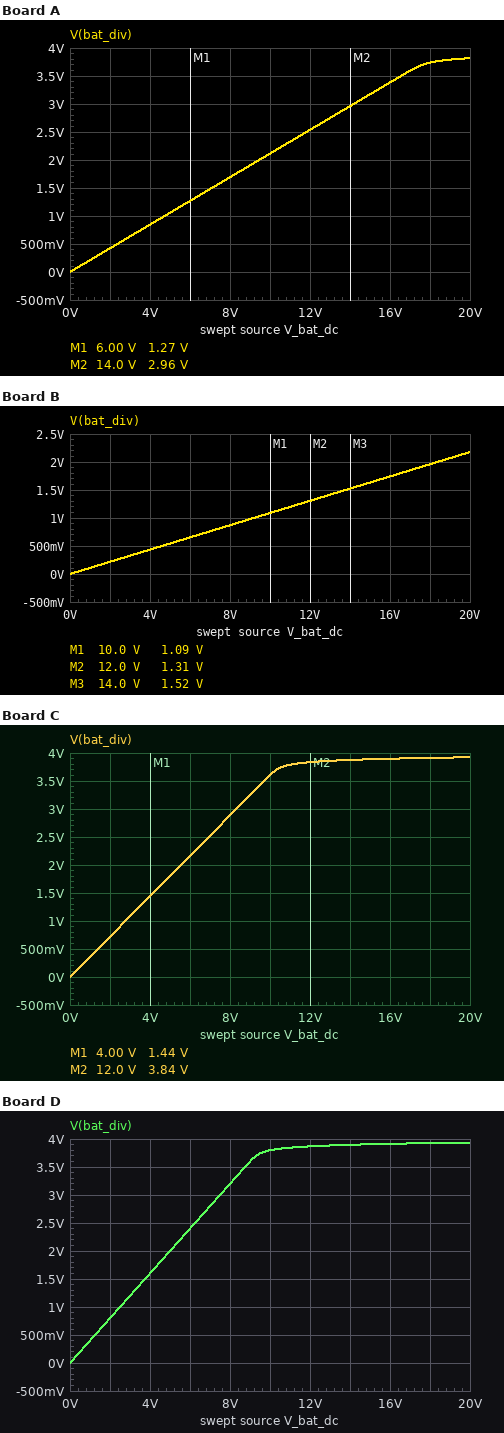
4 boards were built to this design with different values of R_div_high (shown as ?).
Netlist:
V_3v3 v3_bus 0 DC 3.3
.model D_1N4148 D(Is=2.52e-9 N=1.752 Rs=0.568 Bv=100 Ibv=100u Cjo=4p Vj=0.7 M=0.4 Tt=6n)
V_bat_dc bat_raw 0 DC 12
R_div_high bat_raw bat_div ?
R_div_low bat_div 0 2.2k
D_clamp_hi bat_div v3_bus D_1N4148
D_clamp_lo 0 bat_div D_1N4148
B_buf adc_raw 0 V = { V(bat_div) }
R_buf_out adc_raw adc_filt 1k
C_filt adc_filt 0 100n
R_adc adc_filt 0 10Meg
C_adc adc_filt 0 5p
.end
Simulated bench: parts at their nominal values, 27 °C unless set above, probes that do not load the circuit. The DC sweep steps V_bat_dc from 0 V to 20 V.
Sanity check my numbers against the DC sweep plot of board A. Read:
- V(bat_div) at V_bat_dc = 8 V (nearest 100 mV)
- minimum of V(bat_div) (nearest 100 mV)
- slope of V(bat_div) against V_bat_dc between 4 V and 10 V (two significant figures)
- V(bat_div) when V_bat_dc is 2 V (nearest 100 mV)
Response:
1.7 V
0 V
0.21 V/V
400 mV
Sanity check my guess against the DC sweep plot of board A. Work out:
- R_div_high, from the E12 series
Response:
8.2 kΩ
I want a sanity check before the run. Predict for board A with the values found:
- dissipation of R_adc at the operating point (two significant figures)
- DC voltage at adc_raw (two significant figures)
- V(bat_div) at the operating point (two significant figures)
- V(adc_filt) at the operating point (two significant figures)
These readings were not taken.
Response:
640 nW
2.5 V
2.5 V
2.5 V
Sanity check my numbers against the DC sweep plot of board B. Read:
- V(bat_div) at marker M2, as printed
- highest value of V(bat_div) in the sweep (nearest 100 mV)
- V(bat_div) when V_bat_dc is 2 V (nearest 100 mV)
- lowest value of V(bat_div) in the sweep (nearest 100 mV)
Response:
1.31 V
2.2 V
200 mV
0 V
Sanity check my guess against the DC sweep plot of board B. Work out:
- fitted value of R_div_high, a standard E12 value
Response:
18 kΩ
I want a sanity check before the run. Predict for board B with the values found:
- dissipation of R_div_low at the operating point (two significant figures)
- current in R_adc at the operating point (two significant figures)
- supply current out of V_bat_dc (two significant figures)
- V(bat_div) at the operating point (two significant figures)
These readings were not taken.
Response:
780 µW
130 nA
590 µA
1.3 V
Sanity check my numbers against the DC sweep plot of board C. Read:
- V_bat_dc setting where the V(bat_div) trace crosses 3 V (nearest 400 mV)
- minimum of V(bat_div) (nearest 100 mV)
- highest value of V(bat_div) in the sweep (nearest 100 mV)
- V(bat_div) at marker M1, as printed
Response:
8.4 V
0 V
3.9 V
1.44 V
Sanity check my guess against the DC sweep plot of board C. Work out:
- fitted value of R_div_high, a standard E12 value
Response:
3.9 kΩ
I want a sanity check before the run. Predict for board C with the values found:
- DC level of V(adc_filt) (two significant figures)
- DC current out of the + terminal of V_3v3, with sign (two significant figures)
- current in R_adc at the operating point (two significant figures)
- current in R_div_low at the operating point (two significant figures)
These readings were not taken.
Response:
3.8 V
-350 µA
380 nA
1.7 mA
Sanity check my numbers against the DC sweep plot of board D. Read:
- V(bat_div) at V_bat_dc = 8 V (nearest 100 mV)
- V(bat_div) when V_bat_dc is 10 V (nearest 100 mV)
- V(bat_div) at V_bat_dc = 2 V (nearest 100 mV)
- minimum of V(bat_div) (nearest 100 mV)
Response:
3.2 V
3.8 V
800 mV
0 V
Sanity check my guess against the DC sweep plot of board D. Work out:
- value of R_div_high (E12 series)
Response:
3.3 kΩ
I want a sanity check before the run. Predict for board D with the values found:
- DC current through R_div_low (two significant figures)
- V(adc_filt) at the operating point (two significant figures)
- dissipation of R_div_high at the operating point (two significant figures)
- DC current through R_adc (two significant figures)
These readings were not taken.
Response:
1.8 mA
3.9 V
20 mW
390 nA
